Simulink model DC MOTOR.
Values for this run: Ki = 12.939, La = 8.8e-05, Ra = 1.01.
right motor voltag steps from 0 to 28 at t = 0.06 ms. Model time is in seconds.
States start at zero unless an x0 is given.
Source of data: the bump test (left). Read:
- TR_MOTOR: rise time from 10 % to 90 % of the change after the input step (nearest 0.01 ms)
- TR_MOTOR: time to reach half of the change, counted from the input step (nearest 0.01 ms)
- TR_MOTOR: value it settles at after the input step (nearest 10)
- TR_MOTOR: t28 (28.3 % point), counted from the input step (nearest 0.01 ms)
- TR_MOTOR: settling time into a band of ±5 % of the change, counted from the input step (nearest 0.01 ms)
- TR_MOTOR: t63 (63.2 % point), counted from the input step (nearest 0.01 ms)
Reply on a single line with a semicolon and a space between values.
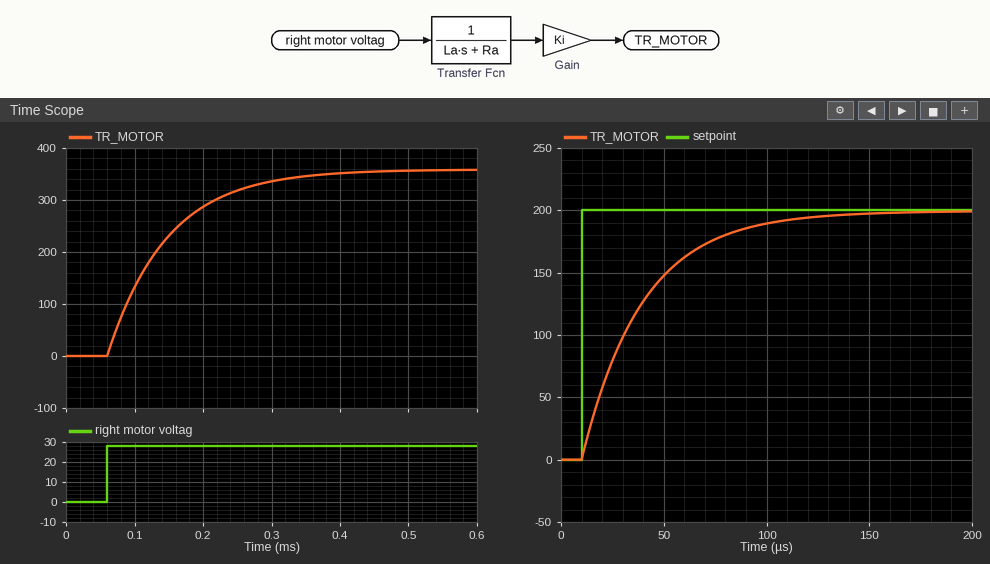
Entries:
0.19 ms; 0.06 ms; 360; 0.03 ms; 0.26 ms; 0.09 ms
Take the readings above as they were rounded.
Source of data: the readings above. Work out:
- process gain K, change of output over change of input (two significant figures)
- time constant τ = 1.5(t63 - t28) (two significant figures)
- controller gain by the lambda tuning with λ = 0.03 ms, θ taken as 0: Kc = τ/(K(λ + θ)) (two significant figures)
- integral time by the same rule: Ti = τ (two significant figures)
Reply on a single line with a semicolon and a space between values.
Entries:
13; 0.090 ms; 0.23; 0.090 ms
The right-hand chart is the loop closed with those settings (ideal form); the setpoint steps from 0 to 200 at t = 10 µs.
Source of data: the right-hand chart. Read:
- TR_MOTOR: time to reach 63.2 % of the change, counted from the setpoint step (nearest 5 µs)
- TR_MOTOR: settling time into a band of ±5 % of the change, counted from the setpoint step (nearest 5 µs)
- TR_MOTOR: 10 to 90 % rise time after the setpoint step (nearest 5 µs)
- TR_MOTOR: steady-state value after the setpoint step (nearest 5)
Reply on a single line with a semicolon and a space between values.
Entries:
30 µs; 90 µs; 65 µs; 200
